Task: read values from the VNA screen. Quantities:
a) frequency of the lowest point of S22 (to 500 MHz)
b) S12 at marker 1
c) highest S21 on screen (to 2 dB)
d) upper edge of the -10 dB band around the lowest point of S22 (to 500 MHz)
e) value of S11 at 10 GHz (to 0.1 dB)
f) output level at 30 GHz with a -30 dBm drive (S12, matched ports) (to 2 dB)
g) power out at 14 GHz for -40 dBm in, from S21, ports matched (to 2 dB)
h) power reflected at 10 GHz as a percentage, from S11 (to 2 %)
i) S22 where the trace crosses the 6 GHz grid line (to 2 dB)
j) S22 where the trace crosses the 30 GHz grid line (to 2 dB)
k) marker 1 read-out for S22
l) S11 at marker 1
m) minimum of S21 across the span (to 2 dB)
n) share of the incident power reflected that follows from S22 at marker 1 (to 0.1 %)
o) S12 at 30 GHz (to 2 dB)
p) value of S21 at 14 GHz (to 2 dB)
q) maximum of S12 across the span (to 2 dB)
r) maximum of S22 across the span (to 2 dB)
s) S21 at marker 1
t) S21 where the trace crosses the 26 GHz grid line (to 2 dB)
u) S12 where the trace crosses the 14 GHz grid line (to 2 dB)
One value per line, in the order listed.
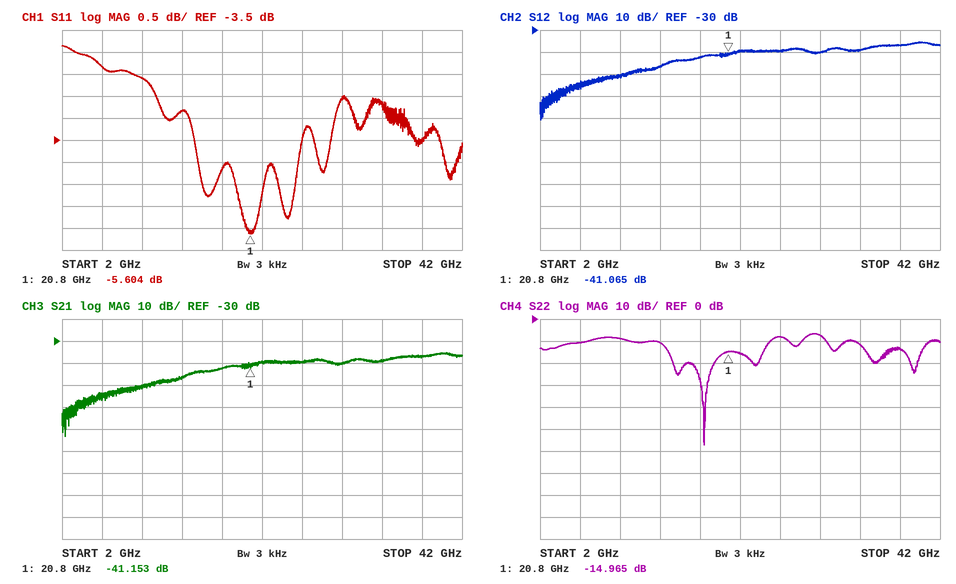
18.5 GHz
-41.065 dB
-36 dB
25.0 GHz
-2.1 dB
-70 dBm
-86 dBm
62 %
-10 dB
-8 dB
-14.965 dB
-5.604 dB
-74 dB
3.2 %
-40 dB
-46 dB
-36 dB
-6 dB
-41.153 dB
-40 dB
-46 dB
